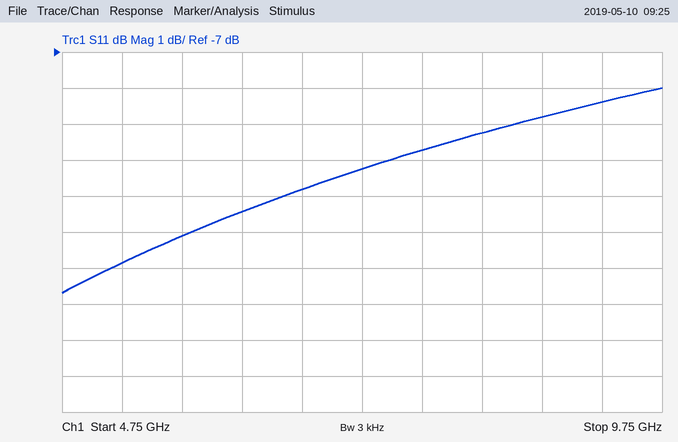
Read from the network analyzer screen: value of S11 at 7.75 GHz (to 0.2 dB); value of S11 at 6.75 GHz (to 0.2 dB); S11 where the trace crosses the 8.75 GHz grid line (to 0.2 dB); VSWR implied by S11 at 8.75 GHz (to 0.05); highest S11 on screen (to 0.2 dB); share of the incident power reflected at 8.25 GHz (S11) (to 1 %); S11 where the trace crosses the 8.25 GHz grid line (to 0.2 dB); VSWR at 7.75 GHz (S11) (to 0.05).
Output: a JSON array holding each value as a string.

["-9.8 dB", "-10.8 dB", "-8.8 dB", "2.15", "-8.0 dB", "12 %", "-9.2 dB", "1.95"]
